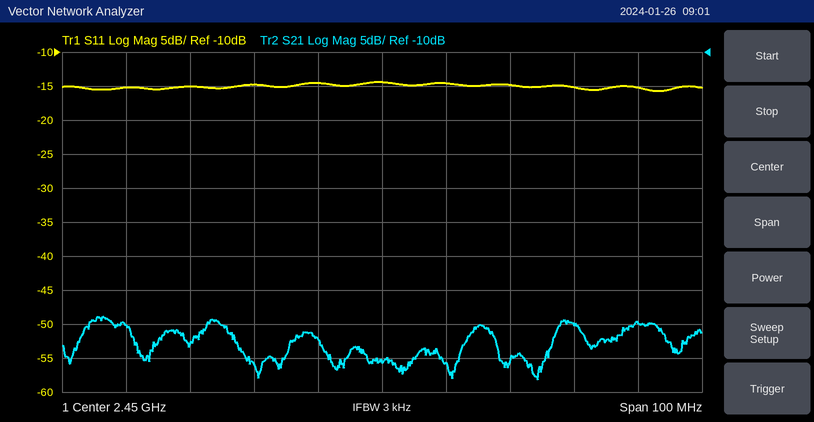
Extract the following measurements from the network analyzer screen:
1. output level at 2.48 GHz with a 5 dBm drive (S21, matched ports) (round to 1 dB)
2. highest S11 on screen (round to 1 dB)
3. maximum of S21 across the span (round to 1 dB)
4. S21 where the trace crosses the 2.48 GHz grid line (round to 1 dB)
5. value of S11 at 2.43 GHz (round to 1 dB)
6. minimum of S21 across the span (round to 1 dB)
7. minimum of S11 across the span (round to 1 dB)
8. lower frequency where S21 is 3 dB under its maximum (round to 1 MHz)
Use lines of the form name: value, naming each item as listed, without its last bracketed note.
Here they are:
output level at 2.48 GHz with a 5 dBm drive (S21, matched ports): -45 dBm
highest S11 on screen: -14 dB
maximum of S21 across the span: -49 dB
S21 where the trace crosses the 2.48 GHz grid line: -50 dB
value of S11 at 2.43 GHz: -15 dB
minimum of S21 across the span: -58 dB
minimum of S11 across the span: -16 dB
lower frequency where S21 is 3 dB under its maximum: 2.403 GHz
